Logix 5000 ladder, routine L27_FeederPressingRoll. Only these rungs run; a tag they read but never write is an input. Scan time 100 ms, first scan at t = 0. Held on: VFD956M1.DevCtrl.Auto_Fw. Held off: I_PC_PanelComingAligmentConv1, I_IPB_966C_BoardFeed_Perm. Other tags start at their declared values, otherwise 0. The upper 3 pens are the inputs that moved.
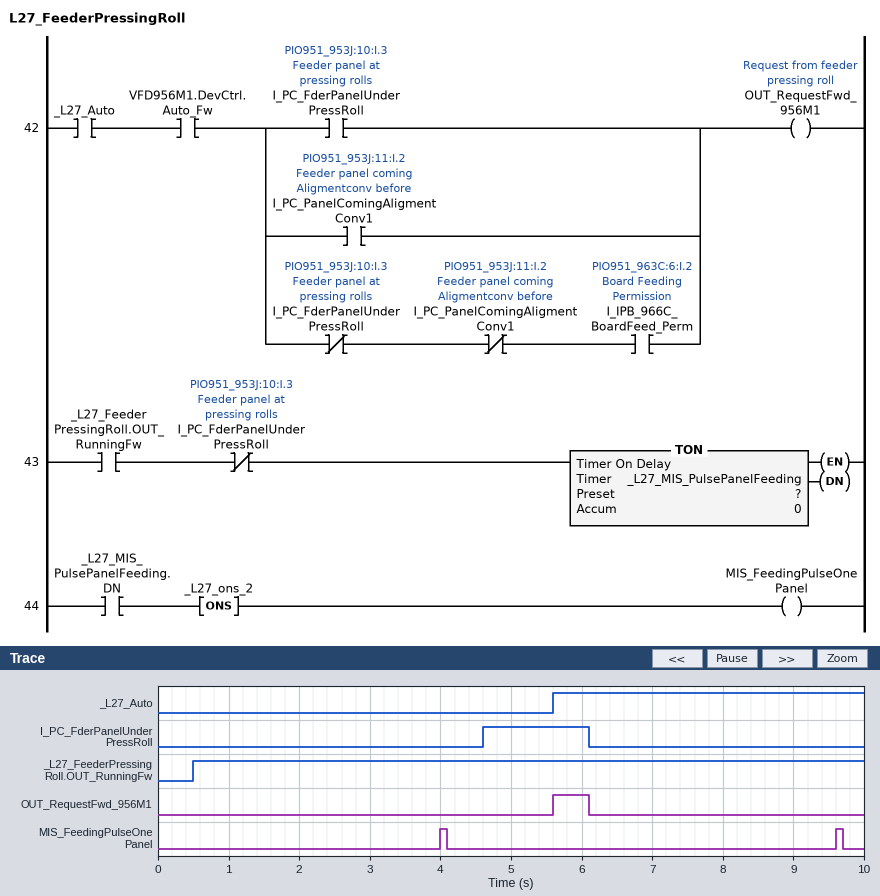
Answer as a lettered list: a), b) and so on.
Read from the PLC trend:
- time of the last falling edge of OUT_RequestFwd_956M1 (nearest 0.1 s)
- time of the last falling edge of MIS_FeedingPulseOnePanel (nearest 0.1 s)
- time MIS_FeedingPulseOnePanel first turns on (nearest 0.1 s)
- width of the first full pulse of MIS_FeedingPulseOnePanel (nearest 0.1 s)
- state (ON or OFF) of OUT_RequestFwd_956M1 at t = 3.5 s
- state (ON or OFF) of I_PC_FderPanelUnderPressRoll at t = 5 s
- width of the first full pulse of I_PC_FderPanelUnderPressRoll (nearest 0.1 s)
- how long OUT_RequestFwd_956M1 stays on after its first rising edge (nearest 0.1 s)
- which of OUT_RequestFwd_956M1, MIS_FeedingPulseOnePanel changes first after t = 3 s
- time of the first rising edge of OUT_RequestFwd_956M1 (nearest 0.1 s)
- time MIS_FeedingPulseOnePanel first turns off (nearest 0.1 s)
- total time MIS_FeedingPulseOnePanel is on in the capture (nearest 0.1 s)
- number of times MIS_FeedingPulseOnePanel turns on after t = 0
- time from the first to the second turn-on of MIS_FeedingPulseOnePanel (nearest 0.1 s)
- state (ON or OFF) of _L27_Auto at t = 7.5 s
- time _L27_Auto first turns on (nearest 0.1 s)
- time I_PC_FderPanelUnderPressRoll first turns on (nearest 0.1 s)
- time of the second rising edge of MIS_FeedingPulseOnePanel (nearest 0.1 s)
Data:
a) 6.1 s
b) 9.7 s
c) 4.0 s
d) 0.1 s
e) OFF
f) ON
g) 1.5 s
h) 0.5 s
i) MIS_FeedingPulseOnePanel
j) 5.6 s
k) 4.1 s
l) 0.2 s
m) 2
n) 5.6 s
o) ON
p) 5.6 s
q) 4.6 s
r) 9.6 s
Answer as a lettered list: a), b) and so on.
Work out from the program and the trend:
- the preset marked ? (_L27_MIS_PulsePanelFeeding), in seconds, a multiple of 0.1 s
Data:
a) 3.5 s
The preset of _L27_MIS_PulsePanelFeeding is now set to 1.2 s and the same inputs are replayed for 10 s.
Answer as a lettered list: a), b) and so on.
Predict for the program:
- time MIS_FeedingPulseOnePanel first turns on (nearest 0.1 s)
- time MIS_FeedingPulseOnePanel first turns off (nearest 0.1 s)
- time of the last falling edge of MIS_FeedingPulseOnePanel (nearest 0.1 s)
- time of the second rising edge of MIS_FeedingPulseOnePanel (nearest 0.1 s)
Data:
a) 1.7 s
b) 1.8 s
c) 7.4 s
d) 7.3 s
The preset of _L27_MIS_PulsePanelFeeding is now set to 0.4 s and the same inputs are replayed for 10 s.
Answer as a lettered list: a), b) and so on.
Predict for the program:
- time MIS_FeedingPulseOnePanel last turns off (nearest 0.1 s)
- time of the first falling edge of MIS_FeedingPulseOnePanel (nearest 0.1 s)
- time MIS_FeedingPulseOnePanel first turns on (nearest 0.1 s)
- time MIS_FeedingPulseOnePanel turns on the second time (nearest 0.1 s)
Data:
a) 6.6 s
b) 1.0 s
c) 0.9 s
d) 6.5 s
